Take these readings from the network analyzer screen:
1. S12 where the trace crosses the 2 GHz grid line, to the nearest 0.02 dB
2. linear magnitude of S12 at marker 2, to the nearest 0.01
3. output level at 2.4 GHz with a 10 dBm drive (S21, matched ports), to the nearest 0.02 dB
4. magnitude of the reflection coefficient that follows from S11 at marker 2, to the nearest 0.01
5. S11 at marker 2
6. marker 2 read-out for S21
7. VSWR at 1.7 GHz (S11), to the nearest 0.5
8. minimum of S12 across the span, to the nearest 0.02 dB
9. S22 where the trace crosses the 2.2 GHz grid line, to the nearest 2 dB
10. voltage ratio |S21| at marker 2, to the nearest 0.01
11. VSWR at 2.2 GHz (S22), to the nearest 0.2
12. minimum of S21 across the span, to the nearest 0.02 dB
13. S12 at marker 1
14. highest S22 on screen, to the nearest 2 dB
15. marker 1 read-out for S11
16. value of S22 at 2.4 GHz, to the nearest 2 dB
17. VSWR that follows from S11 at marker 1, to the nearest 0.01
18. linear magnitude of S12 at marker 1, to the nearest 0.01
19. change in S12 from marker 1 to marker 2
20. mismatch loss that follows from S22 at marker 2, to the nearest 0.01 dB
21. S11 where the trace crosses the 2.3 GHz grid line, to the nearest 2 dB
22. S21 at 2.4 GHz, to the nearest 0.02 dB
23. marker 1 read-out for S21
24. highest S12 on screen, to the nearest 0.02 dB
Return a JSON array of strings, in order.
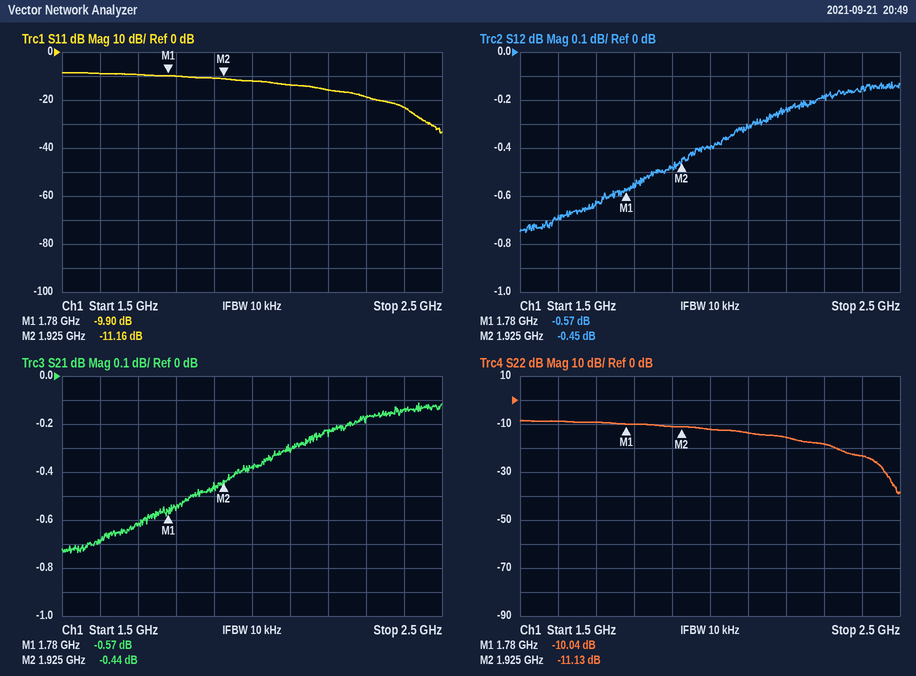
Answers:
["-0.40 dB", "0.95", "9.86 dBm", "0.28", "-11.16 dB", "-0.44 dB", "2.0", "-0.76 dB", "-16 dB", "0.95", "1.4", "-0.74 dB", "-0.57 dB", "-8 dB", "-9.90 dB", "-24 dB", "1.94", "0.94", "0.12 dB", "0.35 dB", "-18 dB", "-0.14 dB", "-0.57 dB", "-0.12 dB"]
